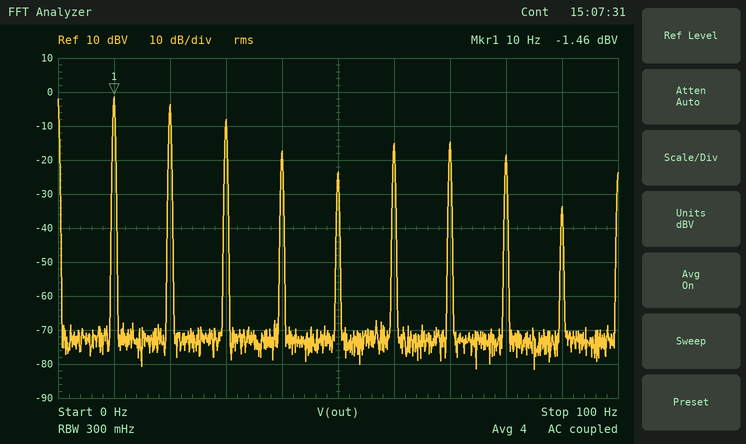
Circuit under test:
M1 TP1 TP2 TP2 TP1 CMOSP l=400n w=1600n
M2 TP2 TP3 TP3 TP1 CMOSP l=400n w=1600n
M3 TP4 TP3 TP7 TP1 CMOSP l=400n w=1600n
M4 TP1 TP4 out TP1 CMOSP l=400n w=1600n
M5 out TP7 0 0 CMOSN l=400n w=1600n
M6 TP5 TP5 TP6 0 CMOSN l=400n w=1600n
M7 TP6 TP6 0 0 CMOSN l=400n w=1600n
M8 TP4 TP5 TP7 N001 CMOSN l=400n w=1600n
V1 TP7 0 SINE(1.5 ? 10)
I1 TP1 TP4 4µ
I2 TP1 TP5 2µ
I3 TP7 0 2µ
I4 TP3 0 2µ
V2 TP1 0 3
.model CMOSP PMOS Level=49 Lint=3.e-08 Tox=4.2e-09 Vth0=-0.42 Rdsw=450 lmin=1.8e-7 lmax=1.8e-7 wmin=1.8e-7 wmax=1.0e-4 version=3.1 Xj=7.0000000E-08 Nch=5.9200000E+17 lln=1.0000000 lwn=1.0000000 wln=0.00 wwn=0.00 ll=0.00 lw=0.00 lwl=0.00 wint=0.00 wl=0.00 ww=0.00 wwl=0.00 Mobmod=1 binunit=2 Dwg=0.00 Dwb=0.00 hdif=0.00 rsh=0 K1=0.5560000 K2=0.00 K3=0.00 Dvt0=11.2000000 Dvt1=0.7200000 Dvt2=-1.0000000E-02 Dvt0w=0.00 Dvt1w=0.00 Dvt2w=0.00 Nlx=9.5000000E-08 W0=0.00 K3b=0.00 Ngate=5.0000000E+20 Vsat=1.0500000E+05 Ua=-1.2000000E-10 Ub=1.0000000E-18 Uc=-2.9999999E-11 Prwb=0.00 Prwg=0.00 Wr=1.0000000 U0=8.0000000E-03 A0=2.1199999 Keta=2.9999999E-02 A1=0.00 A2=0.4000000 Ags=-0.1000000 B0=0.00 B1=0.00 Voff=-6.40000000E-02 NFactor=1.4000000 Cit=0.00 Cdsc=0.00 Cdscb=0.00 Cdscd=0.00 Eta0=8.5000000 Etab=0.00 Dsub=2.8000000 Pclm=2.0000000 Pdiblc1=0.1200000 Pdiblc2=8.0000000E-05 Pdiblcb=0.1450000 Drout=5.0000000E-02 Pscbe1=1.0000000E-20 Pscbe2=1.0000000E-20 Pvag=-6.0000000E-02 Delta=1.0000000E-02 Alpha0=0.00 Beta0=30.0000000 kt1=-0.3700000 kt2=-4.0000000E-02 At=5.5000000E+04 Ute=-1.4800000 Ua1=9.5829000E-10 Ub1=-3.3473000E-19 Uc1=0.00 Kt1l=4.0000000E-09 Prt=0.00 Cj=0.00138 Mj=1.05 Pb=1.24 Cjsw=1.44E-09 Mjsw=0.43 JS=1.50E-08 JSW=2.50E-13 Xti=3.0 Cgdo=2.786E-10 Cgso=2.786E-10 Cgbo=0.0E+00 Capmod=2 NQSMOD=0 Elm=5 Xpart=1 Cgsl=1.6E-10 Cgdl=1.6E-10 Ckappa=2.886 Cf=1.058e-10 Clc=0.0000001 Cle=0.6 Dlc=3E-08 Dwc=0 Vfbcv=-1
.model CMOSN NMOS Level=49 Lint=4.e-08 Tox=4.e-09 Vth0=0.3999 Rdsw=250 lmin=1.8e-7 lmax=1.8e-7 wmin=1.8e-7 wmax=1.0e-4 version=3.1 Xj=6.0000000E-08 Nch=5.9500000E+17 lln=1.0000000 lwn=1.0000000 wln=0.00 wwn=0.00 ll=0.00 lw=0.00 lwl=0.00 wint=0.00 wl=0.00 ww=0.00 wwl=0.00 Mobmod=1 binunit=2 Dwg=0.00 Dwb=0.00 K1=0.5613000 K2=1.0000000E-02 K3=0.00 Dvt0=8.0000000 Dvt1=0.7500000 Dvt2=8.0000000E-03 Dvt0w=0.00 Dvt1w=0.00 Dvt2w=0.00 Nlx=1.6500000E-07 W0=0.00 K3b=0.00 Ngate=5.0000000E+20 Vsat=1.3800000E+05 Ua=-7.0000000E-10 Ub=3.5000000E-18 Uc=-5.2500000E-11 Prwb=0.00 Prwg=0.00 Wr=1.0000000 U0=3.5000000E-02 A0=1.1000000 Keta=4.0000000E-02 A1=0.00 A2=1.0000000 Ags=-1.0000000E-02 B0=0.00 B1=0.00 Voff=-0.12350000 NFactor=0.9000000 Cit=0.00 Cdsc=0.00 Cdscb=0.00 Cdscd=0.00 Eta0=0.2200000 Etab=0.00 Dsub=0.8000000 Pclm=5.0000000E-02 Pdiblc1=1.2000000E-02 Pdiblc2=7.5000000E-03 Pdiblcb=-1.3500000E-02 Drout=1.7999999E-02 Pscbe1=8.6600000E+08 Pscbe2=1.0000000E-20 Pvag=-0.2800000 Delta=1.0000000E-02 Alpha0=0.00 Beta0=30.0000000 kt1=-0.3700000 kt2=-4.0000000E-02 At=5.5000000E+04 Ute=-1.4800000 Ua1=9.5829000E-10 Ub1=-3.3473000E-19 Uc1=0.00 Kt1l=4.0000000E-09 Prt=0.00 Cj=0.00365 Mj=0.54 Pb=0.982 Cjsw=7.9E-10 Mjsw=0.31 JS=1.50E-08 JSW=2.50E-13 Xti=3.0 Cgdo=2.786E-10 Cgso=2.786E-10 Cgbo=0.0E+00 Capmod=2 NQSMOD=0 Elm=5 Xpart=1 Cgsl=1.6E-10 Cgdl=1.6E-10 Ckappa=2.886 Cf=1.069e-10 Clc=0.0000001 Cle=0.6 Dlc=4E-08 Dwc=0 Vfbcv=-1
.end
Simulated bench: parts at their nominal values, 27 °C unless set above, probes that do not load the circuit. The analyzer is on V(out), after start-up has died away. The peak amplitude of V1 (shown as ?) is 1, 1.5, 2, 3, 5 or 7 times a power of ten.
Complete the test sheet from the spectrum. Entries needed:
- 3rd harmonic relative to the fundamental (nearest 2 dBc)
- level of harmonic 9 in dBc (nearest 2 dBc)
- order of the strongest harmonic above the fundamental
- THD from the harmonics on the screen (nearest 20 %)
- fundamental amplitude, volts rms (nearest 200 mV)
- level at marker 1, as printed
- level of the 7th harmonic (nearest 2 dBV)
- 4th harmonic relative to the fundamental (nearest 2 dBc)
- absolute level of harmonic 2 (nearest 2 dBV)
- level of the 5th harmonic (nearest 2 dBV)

-6 dBc
-32 dBc
2
100 %
800 mV
-1.46 dBV
-14 dBV
-16 dBc
-4 dBV
-24 dBV
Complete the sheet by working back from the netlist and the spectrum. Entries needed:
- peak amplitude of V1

1 V
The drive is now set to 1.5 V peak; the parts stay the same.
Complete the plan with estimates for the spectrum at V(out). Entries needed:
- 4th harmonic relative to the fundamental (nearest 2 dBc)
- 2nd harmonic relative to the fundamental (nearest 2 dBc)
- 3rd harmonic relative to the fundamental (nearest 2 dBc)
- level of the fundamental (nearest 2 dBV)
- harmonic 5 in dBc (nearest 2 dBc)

-12 dBc
-6 dBc
-32 dBc
2 dBV
-14 dBc
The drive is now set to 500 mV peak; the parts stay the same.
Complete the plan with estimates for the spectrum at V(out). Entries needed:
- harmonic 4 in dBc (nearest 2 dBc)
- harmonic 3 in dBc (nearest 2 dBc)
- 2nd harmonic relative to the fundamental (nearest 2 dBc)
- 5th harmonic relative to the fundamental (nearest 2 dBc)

-34 dBc
-22 dBc
-12 dBc
-44 dBc
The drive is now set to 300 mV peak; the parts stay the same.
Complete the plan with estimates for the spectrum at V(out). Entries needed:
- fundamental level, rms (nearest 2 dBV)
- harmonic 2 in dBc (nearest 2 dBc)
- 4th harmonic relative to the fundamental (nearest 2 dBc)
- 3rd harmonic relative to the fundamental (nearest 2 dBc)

-66 dBV
-16 dBc
-48 dBc
-32 dBc
